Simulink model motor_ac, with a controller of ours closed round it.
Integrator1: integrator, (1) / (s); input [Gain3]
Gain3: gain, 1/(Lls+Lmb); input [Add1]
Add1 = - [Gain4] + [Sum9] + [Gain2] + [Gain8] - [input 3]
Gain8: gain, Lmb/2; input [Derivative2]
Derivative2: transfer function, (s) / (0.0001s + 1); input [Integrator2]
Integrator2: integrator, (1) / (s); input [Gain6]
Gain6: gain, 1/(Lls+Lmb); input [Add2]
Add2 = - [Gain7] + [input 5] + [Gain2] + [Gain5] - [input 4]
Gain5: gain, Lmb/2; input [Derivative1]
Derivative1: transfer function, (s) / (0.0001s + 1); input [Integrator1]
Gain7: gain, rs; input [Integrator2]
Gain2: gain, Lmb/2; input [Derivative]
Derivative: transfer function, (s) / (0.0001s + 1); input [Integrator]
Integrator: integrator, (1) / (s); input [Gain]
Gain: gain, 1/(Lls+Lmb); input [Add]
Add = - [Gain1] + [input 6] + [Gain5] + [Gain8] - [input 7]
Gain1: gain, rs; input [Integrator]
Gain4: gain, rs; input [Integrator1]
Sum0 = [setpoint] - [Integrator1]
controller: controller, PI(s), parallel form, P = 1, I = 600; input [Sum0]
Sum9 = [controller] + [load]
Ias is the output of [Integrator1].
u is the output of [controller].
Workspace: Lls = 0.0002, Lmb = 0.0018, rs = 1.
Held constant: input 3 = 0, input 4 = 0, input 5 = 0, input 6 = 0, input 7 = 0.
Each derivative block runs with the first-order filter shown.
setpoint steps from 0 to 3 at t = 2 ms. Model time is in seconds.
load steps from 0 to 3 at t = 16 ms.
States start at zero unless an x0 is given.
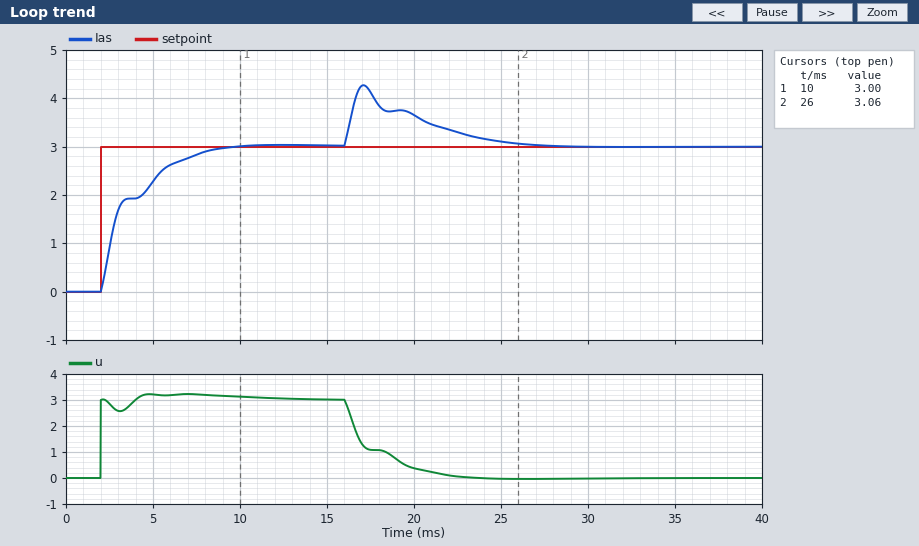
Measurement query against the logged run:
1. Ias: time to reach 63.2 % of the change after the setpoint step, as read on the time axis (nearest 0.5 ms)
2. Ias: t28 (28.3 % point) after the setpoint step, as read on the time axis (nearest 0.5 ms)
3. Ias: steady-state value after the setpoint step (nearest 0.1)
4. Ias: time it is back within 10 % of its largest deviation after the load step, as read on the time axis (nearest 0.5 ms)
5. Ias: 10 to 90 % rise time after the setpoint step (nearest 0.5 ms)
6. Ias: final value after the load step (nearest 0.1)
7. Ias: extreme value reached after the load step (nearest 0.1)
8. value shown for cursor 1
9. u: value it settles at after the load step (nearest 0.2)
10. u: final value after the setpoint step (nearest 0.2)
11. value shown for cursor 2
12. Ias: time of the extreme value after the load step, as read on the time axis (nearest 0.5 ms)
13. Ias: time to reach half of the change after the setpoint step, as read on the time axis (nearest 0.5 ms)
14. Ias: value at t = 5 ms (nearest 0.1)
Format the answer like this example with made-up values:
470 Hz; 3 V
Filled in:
3.5 ms; 2.5 ms; 3.0; 24.5 ms; 4.5 ms; 3.0; 4.3; 3.00; 0.0; 3.0; 3.06; 17.0 ms; 3.0 ms; 2.3
